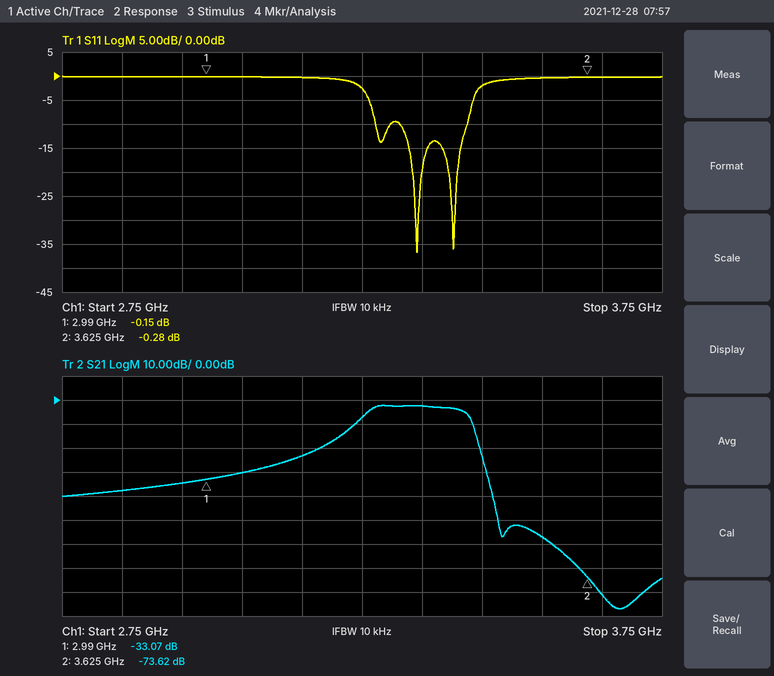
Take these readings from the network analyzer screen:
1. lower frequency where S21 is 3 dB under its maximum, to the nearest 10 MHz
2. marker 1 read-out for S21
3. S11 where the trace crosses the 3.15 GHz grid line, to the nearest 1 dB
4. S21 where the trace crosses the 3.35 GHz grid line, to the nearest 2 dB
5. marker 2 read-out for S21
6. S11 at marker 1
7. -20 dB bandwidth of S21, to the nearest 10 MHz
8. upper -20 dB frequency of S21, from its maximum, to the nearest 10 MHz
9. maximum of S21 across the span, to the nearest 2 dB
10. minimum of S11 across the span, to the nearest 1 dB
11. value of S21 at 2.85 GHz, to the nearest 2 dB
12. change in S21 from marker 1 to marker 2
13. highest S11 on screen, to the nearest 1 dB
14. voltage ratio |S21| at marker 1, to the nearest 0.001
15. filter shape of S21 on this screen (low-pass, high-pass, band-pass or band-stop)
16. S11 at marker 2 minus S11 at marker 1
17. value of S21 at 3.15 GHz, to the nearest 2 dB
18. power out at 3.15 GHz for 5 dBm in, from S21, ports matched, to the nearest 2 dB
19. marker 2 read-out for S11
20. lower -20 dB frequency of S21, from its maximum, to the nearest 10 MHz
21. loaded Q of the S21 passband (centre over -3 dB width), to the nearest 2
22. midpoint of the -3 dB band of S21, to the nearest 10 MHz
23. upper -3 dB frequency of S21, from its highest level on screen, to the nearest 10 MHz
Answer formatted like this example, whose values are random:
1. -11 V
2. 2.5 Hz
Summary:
1. 3.26 GHz
2. -33.07 dB
3. 0 dB
4. -2 dB
5. -73.62 dB
6. -0.15 dB
7. 290 MHz
8. 3.45 GHz
9. -2 dB
10. -37 dB
11. -38 dB
12. -40.55 dB
13. 0 dB
14. 0.022
15. band-pass
16. -0.13 dB
17. -24 dB
18. -18 dBm
19. -0.28 dB
20. 3.16 GHz
21. 20
22. 3.34 GHz
23. 3.42 GHz
